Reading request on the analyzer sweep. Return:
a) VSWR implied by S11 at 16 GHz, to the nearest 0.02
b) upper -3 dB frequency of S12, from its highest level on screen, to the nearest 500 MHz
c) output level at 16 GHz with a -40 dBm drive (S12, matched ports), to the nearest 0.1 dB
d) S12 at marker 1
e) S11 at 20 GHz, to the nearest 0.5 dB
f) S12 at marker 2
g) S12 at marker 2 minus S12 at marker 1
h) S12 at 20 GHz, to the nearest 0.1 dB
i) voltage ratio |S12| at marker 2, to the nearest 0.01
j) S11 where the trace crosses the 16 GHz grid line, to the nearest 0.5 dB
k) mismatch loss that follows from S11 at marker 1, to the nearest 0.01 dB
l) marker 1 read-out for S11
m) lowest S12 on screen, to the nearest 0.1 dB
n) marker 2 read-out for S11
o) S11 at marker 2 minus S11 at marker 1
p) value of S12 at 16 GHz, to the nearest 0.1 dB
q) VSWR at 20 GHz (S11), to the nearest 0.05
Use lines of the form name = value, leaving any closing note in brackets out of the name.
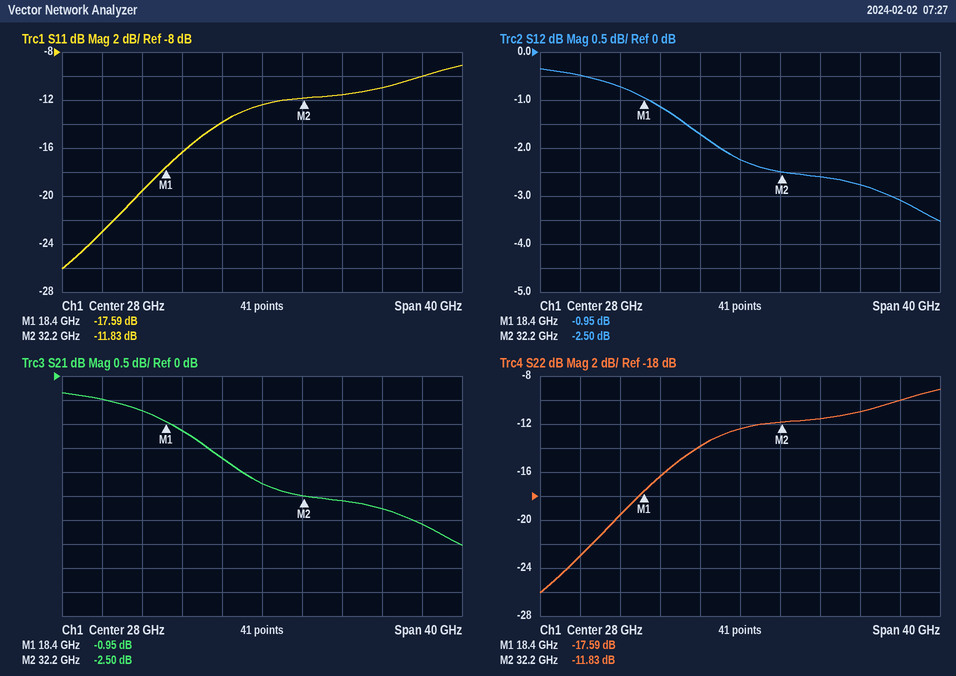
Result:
VSWR implied by S11 at 16 GHz, to the nearest 0.02 = 1.24
upper -3 dB frequency of S12, from its highest level on screen, to the nearest 500 MHz = 46.5 GHz
output level at 16 GHz with a -40 dBm drive (S12, matched ports), to the nearest 0.1 dB = -40.7 dBm
S12 at marker 1 = -0.95 dB
S11 at 20 GHz, to the nearest 0.5 dB = -16.5 dB
S12 at marker 2 = -2.50 dB
S12 at marker 2 minus S12 at marker 1 = -1.55 dB
S12 at 20 GHz, to the nearest 0.1 dB = -1.1 dB
voltage ratio |S12| at marker 2, to the nearest 0.01 = 0.75
S11 where the trace crosses the 16 GHz grid line, to the nearest 0.5 dB = -19.5 dB
mismatch loss that follows from S11 at marker 1, to the nearest 0.01 dB = 0.08 dB
marker 1 read-out for S11 = -17.59 dB
lowest S12 on screen, to the nearest 0.1 dB = -3.5 dB
marker 2 read-out for S11 = -11.83 dB
S11 at marker 2 minus S11 at marker 1 = 5.76 dB
value of S12 at 16 GHz, to the nearest 0.1 dB = -0.7 dB
VSWR at 20 GHz (S11), to the nearest 0.05 = 1.35
